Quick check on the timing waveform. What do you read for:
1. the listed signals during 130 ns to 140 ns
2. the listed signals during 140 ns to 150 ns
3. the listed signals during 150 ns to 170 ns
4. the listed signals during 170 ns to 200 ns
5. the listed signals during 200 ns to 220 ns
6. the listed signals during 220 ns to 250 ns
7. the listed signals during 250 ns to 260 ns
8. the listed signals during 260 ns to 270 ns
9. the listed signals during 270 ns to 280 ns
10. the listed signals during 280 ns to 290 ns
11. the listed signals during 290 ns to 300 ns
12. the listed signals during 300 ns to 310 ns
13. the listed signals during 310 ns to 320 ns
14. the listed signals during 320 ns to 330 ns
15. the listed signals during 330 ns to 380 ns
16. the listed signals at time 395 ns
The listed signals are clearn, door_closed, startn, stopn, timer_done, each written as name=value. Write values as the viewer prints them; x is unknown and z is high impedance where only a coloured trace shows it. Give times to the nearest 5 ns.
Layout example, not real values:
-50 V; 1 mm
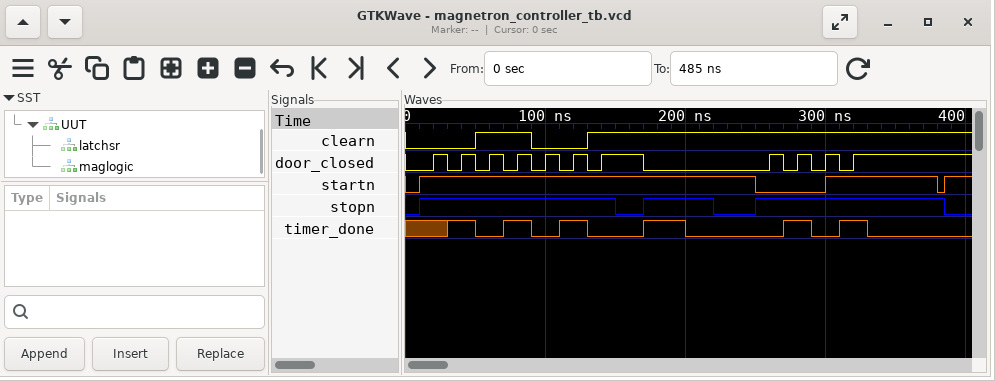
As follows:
clearn=1, door_closed=0, startn=1, stopn=1, timer_done=0; clearn=1, door_closed=1, startn=1, stopn=1, timer_done=0; clearn=1, door_closed=1, startn=1, stopn=0, timer_done=0; clearn=1, door_closed=0, startn=1, stopn=1, timer_done=1; clearn=1, door_closed=0, startn=1, stopn=1, timer_done=0; clearn=1, door_closed=0, startn=1, stopn=0, timer_done=0; clearn=1, door_closed=0, startn=0, stopn=1, timer_done=0; clearn=1, door_closed=1, startn=0, stopn=1, timer_done=0; clearn=1, door_closed=0, startn=0, stopn=1, timer_done=1; clearn=1, door_closed=1, startn=0, stopn=1, timer_done=1; clearn=1, door_closed=0, startn=0, stopn=1, timer_done=0; clearn=1, door_closed=1, startn=1, stopn=1, timer_done=0; clearn=1, door_closed=0, startn=1, stopn=1, timer_done=1; clearn=1, door_closed=1, startn=1, stopn=1, timer_done=1; clearn=1, door_closed=1, startn=1, stopn=1, timer_done=0; clearn=1, door_closed=1, startn=1, stopn=0, timer_done=0
